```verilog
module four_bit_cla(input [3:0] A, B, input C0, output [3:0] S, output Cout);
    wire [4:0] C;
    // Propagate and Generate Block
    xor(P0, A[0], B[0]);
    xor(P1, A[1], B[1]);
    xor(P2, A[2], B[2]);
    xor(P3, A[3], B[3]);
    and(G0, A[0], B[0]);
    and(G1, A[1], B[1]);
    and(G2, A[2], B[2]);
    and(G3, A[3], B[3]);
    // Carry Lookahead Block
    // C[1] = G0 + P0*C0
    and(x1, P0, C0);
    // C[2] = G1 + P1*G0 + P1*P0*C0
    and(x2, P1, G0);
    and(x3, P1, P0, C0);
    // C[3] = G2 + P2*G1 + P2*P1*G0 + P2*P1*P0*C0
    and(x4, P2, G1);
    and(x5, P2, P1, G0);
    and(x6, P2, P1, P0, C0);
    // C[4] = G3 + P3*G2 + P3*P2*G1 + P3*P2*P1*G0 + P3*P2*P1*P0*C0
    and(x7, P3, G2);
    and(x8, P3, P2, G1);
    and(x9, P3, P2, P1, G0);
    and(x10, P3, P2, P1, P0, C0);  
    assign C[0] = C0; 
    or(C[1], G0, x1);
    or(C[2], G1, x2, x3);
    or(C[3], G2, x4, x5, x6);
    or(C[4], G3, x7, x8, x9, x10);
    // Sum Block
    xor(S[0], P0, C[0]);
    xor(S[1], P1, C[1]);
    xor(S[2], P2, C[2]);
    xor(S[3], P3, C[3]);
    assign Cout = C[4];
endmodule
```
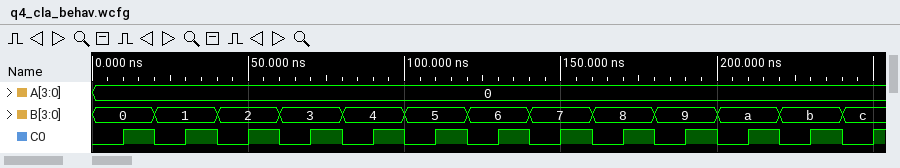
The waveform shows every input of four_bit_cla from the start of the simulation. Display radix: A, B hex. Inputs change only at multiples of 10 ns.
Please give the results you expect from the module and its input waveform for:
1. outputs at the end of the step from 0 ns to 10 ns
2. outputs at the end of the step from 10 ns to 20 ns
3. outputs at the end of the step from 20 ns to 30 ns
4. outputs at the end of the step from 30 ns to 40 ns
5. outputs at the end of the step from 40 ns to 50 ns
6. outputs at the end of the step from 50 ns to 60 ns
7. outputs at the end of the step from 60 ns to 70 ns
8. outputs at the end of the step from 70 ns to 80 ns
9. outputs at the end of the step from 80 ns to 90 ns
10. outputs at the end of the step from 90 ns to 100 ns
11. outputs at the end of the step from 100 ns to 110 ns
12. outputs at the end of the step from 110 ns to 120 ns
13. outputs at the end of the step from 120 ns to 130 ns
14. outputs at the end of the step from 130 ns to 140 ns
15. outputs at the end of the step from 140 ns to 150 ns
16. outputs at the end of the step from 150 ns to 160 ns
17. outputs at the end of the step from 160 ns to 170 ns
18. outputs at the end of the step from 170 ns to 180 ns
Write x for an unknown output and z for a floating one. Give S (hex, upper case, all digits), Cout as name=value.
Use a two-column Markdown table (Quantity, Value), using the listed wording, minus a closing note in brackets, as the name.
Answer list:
| Quantity | Value |
|---|---|
| outputs at the end of the step from 0 ns to 10 ns | S=0, Cout=0 |
| outputs at the end of the step from 10 ns to 20 ns | S=1, Cout=0 |
| outputs at the end of the step from 20 ns to 30 ns | S=1, Cout=0 |
| outputs at the end of the step from 30 ns to 40 ns | S=2, Cout=0 |
| outputs at the end of the step from 40 ns to 50 ns | S=2, Cout=0 |
| outputs at the end of the step from 50 ns to 60 ns | S=3, Cout=0 |
| outputs at the end of the step from 60 ns to 70 ns | S=3, Cout=0 |
| outputs at the end of the step from 70 ns to 80 ns | S=4, Cout=0 |
| outputs at the end of the step from 80 ns to 90 ns | S=4, Cout=0 |
| outputs at the end of the step from 90 ns to 100 ns | S=5, Cout=0 |
| outputs at the end of the step from 100 ns to 110 ns | S=5, Cout=0 |
| outputs at the end of the step from 110 ns to 120 ns | S=6, Cout=0 |
| outputs at the end of the step from 120 ns to 130 ns | S=6, Cout=0 |
| outputs at the end of the step from 130 ns to 140 ns | S=7, Cout=0 |
| outputs at the end of the step from 140 ns to 150 ns | S=7, Cout=0 |
| outputs at the end of the step from 150 ns to 160 ns | S=8, Cout=0 |
| outputs at the end of the step from 160 ns to 170 ns | S=8, Cout=0 |
| outputs at the end of the step from 170 ns to 180 ns | S=9, Cout=0 |
